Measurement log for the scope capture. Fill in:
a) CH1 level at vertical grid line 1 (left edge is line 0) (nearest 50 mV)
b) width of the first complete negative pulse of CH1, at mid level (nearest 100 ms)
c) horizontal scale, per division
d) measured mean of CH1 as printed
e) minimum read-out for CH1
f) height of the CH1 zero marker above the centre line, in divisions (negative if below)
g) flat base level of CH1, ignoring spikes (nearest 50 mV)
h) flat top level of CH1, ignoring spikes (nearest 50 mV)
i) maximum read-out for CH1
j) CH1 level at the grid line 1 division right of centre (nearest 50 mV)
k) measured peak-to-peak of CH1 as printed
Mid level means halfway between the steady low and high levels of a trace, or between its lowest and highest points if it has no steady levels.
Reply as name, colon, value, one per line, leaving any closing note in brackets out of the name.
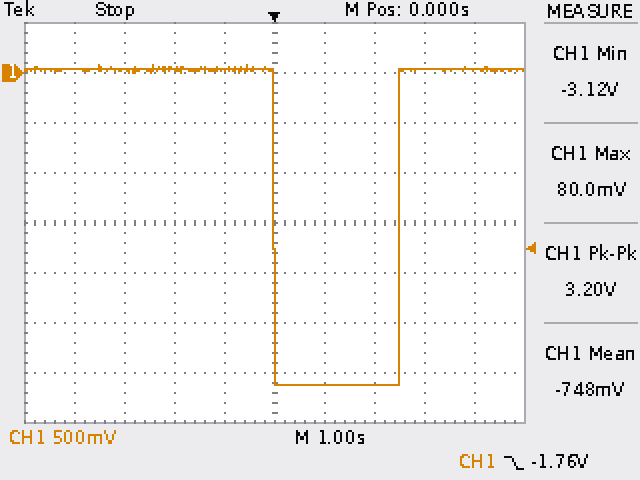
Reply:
CH1 level at vertical grid line 1 (left edge is line 0): 50 mV
width of the first complete negative pulse of CH1, at mid level: 2.5 s
horizontal scale, per division: 1 s
measured mean of CH1 as printed: -748 mV
minimum read-out for CH1: -3.12 V
height of the CH1 zero marker above the centre line, in divisions: +3.0 div
flat base level of CH1, ignoring spikes: -3.10 V
flat top level of CH1, ignoring spikes: 50 mV
maximum read-out for CH1: 80.0 mV
CH1 level at the grid line 1 division right of centre: -3.10 V
measured peak-to-peak of CH1 as printed: 3.20 V
